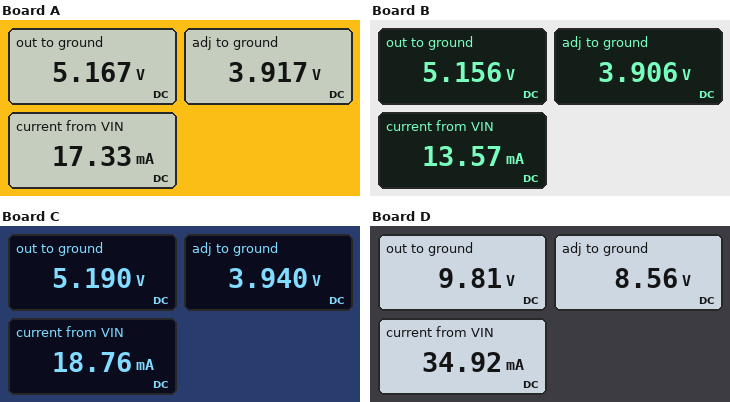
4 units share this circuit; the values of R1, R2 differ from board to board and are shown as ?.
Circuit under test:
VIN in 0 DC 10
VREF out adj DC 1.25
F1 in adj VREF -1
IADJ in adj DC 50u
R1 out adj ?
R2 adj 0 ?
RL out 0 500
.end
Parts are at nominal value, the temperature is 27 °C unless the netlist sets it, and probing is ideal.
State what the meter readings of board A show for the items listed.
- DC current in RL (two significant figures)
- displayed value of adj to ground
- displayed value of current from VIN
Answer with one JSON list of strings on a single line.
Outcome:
["10 mA", "3.917 V", "17.33 mA"]
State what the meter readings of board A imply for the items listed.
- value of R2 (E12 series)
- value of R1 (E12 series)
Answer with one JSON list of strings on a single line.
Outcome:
["560 Ω", "180 Ω"]
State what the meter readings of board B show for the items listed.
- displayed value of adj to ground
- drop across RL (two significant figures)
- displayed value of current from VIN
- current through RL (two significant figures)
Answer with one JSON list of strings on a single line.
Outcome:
["3.906 V", "5.2 V", "13.57 mA", "10 mA"]
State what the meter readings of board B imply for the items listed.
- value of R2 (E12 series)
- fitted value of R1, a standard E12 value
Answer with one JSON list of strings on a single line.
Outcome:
["1.2 kΩ", "390 Ω"]
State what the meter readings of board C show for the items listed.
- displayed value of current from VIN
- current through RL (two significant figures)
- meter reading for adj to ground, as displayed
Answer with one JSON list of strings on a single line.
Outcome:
["18.76 mA", "10 mA", "3.940 V"]
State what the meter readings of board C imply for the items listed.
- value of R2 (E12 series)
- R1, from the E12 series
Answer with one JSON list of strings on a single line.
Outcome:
["470 Ω", "150 Ω"]
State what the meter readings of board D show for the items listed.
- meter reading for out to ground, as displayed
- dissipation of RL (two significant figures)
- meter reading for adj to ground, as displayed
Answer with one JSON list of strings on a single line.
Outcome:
["9.81 V", "190 mW", "8.56 V"]
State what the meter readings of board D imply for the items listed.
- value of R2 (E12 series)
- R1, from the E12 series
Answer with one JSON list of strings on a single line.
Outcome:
["560 Ω", "82 Ω"]
